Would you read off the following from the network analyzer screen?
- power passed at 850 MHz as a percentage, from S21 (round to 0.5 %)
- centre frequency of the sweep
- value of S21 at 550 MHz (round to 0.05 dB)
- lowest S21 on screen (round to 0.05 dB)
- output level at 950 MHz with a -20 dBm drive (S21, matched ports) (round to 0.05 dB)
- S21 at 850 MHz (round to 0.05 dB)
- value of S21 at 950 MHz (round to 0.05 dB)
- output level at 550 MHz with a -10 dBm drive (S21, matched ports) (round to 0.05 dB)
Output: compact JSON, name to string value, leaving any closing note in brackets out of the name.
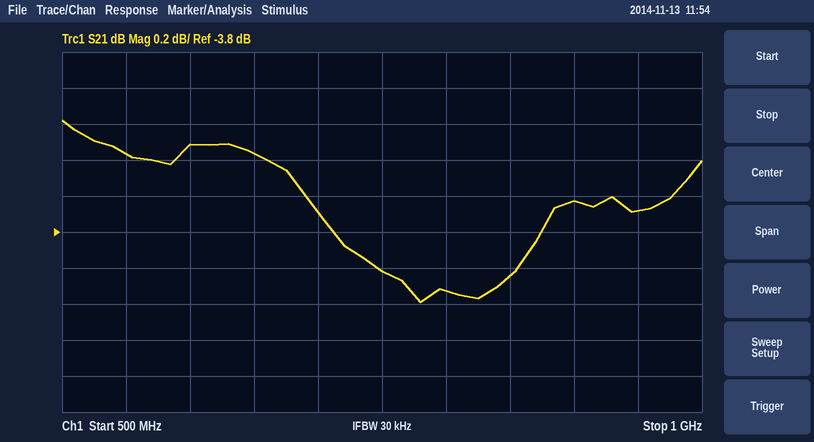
{"power passed at 850 MHz as a percentage, from S21": "39.5 %", "centre frequency of the sweep": "750 MHz", "value of S21 at 550 MHz": "-3.35 dB", "lowest S21 on screen": "-4.20 dB", "output level at 950 MHz with a -20 dBm drive (S21, matched ports)": "-23.70 dBm", "S21 at 850 MHz": "-4.05 dB", "value of S21 at 950 MHz": "-3.70 dB", "output level at 550 MHz with a -10 dBm drive (S21, matched ports)": "-13.35 dBm"}
